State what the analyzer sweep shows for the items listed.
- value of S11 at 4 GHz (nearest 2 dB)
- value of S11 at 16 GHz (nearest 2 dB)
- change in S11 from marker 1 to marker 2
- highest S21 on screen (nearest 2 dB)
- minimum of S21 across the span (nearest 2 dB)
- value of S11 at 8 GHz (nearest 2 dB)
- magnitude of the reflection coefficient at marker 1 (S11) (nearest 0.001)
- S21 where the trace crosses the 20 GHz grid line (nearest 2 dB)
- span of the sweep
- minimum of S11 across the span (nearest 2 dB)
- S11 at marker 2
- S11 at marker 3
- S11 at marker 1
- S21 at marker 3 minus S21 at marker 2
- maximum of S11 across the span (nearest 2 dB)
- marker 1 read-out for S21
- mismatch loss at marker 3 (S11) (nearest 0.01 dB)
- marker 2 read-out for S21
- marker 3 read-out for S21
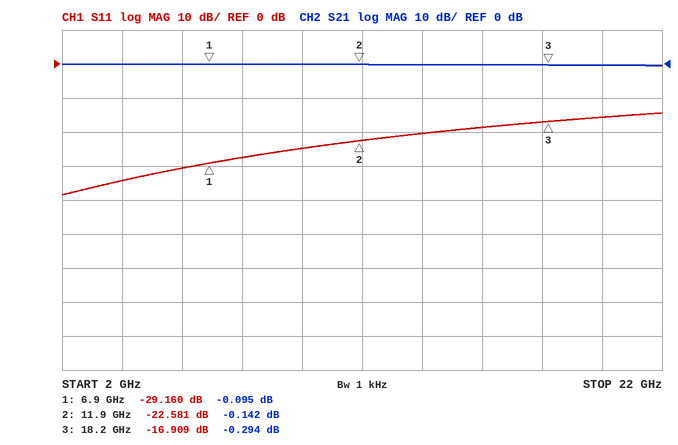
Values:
-34 dB
-18 dB
6.579 dB
0 dB
0 dB
-28 dB
0.035
0 dB
20 GHz
-38 dB
-22.581 dB
-16.909 dB
-29.160 dB
-0.152 dB
-14 dB
-0.095 dB
0.09 dB
-0.142 dB
-0.294 dB
